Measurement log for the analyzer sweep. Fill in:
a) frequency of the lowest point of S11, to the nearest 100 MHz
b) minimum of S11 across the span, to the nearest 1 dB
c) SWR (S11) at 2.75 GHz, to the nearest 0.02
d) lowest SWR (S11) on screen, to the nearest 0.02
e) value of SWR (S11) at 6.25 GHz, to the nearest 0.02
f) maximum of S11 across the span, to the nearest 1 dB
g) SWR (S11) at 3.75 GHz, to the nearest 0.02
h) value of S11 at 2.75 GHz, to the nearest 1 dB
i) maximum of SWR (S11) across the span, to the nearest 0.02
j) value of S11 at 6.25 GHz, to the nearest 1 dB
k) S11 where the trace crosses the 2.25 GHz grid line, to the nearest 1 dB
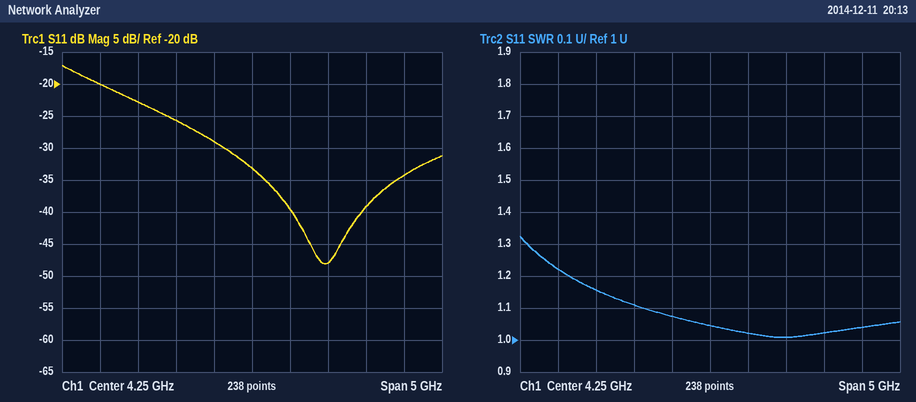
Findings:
5.2 GHz
-48 dB
1.16
1.00
1.04
-17 dB
1.08
-23 dB
1.32
-34 dB
-20 dB
